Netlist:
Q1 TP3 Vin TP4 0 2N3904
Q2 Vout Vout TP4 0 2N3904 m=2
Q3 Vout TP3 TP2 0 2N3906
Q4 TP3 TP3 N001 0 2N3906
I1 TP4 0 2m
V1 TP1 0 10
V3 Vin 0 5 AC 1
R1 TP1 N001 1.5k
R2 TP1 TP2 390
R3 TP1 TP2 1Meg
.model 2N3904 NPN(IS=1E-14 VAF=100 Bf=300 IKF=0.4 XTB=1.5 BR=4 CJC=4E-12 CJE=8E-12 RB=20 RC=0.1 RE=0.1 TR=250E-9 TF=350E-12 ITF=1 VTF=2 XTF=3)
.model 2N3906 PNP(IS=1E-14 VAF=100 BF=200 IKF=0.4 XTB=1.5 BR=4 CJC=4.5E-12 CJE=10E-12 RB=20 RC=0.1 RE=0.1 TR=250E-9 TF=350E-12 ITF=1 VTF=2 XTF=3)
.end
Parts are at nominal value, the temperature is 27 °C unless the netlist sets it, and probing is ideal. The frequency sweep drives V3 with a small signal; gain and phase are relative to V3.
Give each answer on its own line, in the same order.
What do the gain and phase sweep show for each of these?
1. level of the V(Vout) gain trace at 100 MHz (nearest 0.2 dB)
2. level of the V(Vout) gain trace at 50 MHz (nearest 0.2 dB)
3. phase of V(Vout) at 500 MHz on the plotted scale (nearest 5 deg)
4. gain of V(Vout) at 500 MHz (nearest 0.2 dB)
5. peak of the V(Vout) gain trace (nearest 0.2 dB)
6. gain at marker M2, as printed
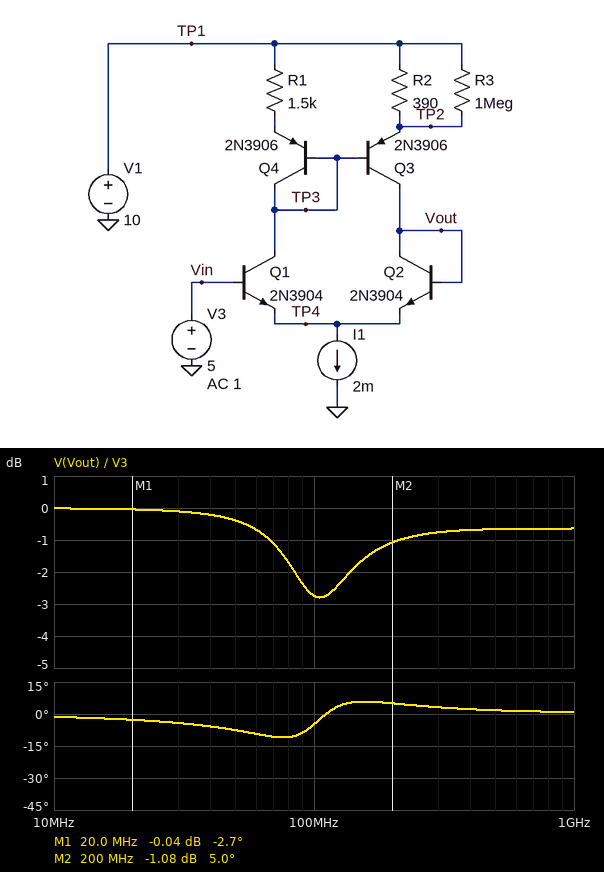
-2.8 dB
-0.4 dB
0 deg
-0.6 dB
0 dB
-1.08 dB
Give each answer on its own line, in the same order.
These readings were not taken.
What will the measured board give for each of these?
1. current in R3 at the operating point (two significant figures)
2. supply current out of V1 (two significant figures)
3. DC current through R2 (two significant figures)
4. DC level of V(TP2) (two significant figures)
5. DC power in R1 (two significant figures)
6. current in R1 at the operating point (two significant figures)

610 nA
2.0 mA
1.6 mA
9.4 V
280 µW
430 µA
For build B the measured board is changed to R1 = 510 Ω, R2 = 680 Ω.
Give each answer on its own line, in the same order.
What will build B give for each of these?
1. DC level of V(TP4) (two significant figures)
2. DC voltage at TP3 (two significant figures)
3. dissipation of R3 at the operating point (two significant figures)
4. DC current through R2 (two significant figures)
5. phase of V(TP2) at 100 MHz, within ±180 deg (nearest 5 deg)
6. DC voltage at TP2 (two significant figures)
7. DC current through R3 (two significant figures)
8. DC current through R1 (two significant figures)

4.3 V
8.8 V
340 nW
860 µA
75 deg
9.4 V
590 nA
1.1 mA
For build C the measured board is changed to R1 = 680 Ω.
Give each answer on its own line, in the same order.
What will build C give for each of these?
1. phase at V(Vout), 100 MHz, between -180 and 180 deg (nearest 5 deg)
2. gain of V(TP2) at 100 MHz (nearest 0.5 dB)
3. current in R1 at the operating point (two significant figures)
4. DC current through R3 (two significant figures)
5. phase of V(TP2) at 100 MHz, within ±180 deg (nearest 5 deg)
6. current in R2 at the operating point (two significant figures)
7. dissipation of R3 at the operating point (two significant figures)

-10 deg
-4.0 dB
740 µA
490 nA
80 deg
1.3 mA
240 nW
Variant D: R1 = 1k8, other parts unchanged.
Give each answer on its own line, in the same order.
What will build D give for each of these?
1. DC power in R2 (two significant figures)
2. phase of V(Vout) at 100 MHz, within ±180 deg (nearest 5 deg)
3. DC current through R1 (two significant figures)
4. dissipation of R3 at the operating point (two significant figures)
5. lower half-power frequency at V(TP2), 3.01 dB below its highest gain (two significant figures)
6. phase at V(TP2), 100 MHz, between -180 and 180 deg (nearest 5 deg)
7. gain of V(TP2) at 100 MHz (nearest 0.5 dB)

1.0 mW
0 deg
370 µA
400 nW
75 MHz
55 deg
0.5 dB
